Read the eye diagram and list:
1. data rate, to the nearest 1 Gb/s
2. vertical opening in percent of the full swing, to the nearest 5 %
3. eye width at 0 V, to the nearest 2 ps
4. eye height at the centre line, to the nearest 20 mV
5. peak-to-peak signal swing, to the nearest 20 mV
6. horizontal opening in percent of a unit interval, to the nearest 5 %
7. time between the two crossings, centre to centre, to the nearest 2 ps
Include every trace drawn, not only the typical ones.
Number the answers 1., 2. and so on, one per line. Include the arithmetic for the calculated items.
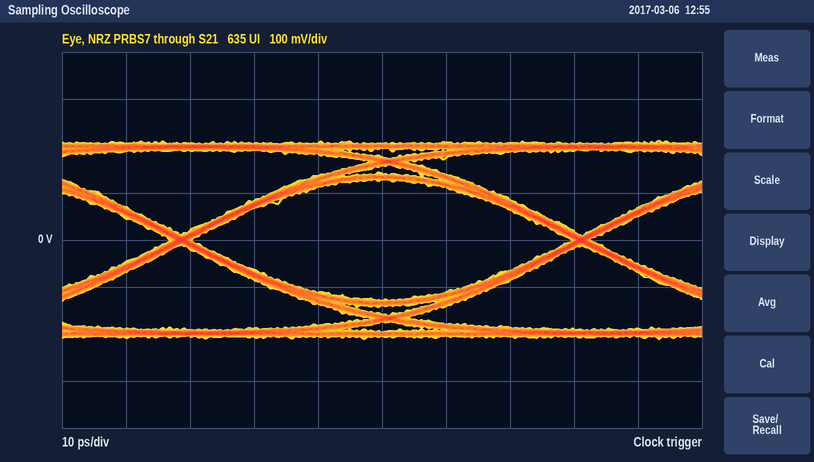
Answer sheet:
1. 16 Gb/s
2. 260 mV / 420 mV ≈ 61.9 %, so 60 % to the nearest 5 %
3. 60 ps
4. 260 mV
5. 420 mV
6. 60 ps / 62 ps ≈ 96.8 %, so 95 % to the nearest 5 %
7. 62 ps
